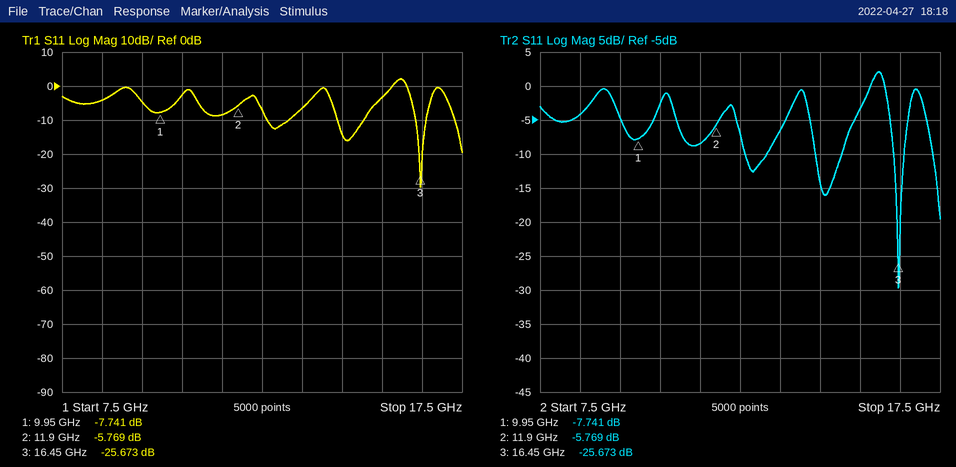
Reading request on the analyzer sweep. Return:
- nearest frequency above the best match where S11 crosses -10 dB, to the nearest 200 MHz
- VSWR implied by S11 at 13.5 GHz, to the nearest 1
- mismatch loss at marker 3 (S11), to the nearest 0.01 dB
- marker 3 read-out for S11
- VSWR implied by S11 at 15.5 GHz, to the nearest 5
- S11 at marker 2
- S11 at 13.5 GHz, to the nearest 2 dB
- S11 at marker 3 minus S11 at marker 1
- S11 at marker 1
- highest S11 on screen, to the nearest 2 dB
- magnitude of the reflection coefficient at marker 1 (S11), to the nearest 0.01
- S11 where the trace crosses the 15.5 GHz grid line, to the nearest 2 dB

16.6 GHz
3
0.01 dB
-25.673 dB
5
-5.769 dB
-6 dB
-17.932 dB
-7.741 dB
2 dB
0.41
-4 dB
